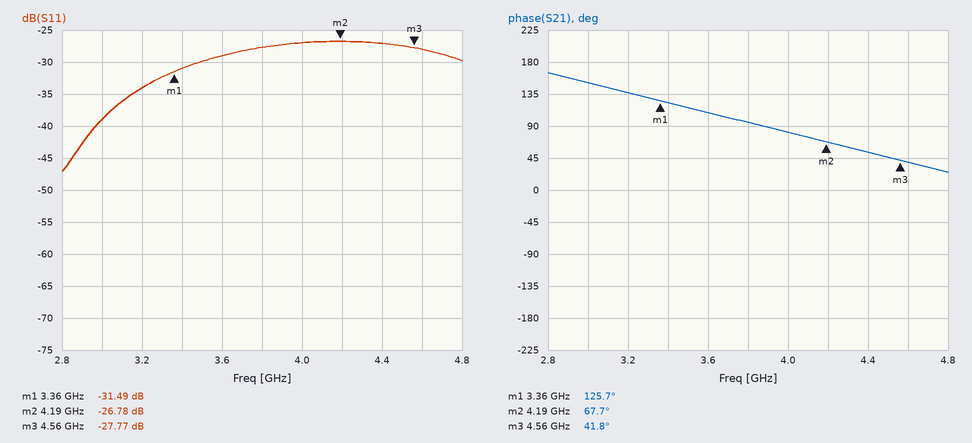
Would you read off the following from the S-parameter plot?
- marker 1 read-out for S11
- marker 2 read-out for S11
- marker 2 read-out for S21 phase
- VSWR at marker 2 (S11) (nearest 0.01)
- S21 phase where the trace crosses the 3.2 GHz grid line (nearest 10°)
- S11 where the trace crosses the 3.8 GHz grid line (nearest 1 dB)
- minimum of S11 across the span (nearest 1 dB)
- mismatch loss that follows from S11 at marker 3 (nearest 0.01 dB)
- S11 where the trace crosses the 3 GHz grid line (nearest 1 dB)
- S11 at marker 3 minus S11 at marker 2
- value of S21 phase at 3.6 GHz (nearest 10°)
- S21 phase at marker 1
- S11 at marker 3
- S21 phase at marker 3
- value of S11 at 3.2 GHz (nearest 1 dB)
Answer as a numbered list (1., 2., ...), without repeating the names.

1. -31.49 dB
2. -26.78 dB
3. 67.7°
4. 1.10
5. 140°
6. -28 dB
7. -47 dB
8. 0.01 dB
9. -39 dB
10. -0.99 dB
11. 110°
12. 125.7°
13. -27.77 dB
14. 41.8°
15. -34 dB
